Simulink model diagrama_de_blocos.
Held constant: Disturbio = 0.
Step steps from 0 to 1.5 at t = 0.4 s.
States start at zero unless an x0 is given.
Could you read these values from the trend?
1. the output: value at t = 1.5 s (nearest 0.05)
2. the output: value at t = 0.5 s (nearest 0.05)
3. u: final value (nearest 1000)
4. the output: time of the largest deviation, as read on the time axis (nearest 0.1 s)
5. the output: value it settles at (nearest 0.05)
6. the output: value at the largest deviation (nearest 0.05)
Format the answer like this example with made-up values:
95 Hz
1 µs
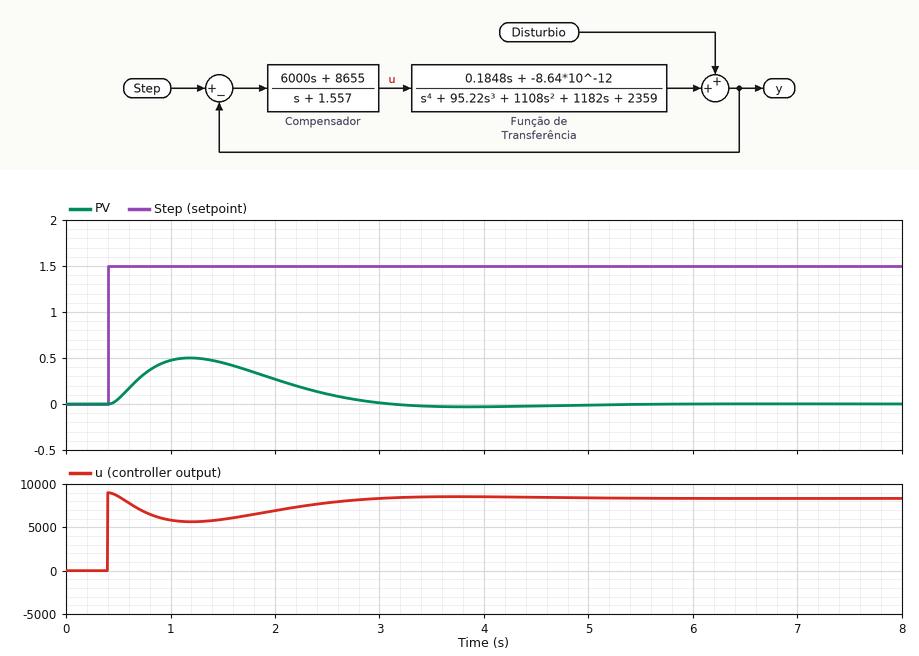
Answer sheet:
0.45
0.05
8000
1.2 s
0.00
0.50
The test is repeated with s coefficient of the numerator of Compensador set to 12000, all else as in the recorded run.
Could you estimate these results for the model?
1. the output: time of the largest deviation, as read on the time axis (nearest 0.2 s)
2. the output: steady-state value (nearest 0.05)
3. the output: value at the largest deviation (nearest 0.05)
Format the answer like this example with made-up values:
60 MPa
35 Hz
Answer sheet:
1.0 s
0.00
0.65
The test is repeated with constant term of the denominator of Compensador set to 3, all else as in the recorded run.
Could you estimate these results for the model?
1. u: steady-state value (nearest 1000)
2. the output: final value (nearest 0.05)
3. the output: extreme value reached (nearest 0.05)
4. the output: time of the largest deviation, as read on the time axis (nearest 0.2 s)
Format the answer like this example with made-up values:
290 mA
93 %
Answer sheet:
4000
0.00
0.35
1.0 s
